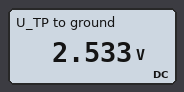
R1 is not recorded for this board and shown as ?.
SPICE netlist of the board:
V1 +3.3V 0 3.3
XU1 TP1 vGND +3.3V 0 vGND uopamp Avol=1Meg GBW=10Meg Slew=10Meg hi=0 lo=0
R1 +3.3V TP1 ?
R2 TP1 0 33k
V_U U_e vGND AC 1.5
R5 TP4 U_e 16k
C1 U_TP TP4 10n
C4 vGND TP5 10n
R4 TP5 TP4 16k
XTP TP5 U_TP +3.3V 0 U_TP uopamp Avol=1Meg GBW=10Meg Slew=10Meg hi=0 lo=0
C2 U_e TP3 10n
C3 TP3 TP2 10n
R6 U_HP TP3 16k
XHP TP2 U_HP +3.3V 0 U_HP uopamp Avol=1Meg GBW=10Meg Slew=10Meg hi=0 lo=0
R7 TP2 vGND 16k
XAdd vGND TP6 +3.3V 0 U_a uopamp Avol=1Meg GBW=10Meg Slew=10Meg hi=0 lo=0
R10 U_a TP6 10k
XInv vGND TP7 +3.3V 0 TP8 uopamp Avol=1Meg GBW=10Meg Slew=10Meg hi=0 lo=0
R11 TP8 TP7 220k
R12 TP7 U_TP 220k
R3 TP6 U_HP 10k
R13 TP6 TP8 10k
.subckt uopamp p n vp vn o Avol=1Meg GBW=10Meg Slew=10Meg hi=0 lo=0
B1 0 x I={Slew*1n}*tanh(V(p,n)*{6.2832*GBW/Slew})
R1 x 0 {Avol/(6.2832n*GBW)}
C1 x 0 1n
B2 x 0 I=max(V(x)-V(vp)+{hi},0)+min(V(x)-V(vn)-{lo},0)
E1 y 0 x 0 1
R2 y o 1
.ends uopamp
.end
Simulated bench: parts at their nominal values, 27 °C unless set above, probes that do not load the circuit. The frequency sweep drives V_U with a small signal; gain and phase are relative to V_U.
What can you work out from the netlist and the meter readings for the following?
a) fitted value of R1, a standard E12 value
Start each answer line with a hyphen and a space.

- 10 kΩ
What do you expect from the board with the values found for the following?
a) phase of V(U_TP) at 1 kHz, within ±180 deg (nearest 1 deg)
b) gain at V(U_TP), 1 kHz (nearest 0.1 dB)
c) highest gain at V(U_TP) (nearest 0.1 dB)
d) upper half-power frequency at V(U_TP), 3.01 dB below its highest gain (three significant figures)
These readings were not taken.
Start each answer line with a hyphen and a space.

- -90 deg
- -6.1 dB
- 0 dB
- 640 Hz
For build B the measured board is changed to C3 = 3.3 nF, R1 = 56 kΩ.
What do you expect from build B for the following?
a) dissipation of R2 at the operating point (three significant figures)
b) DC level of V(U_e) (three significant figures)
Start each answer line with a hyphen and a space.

- 45.4 µW
- 1.22 V
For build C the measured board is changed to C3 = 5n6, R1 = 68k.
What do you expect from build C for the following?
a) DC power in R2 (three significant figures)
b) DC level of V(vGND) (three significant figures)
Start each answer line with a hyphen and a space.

- 35.2 µW
- 1.08 V
